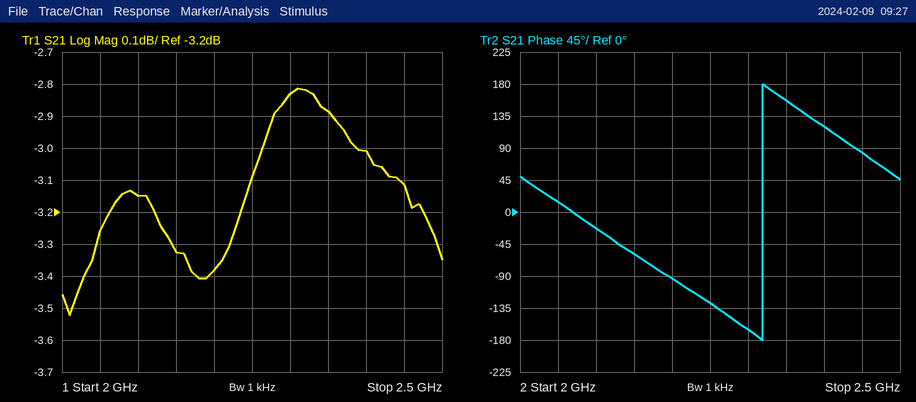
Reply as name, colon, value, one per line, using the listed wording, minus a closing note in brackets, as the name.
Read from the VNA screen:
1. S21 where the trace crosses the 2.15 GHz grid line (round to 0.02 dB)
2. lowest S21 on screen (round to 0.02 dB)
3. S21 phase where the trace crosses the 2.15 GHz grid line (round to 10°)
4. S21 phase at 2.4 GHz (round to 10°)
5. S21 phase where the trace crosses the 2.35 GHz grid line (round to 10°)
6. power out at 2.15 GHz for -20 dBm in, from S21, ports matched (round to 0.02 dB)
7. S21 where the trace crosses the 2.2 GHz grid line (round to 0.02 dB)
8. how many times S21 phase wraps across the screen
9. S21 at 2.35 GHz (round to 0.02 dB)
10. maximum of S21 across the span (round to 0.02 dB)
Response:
S21 where the trace crosses the 2.15 GHz grid line: -3.32 dB
lowest S21 on screen: -3.52 dB
S21 phase where the trace crosses the 2.15 GHz grid line: -60°
S21 phase at 2.4 GHz: 120°
S21 phase where the trace crosses the 2.35 GHz grid line: 160°
power out at 2.15 GHz for -20 dBm in, from S21, ports matched: -23.32 dBm
S21 where the trace crosses the 2.2 GHz grid line: -3.38 dB
how many times S21 phase wraps across the screen: 1
S21 at 2.35 GHz: -2.88 dB
maximum of S21 across the span: -2.82 dB
